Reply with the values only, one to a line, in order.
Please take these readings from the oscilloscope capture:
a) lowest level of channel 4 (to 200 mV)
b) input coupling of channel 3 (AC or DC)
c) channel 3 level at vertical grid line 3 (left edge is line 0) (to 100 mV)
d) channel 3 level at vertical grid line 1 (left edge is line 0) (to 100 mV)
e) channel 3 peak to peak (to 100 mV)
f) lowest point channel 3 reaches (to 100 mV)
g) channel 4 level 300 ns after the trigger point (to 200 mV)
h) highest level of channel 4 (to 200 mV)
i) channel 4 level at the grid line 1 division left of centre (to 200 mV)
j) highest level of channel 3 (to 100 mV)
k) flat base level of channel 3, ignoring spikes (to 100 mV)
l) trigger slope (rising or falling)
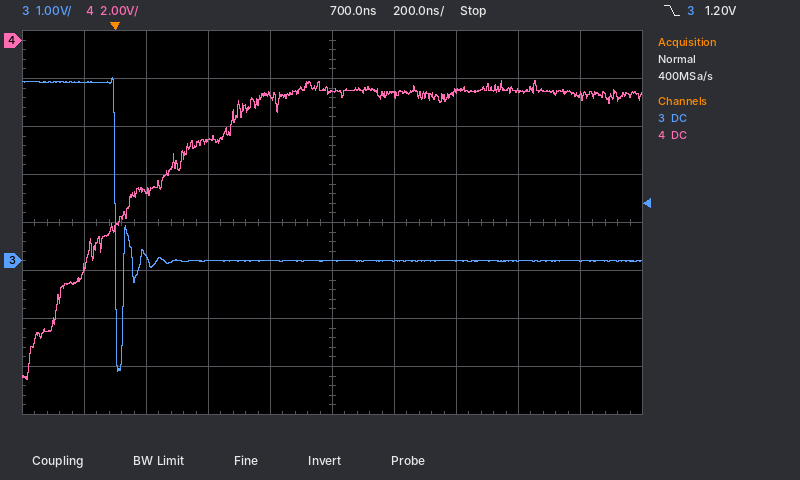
-14.2 V
DC
0.0 V
3.7 V
6.1 V
-2.3 V
-4.2 V
-1.6 V
-2.4 V
3.8 V
0.0 V
falling
